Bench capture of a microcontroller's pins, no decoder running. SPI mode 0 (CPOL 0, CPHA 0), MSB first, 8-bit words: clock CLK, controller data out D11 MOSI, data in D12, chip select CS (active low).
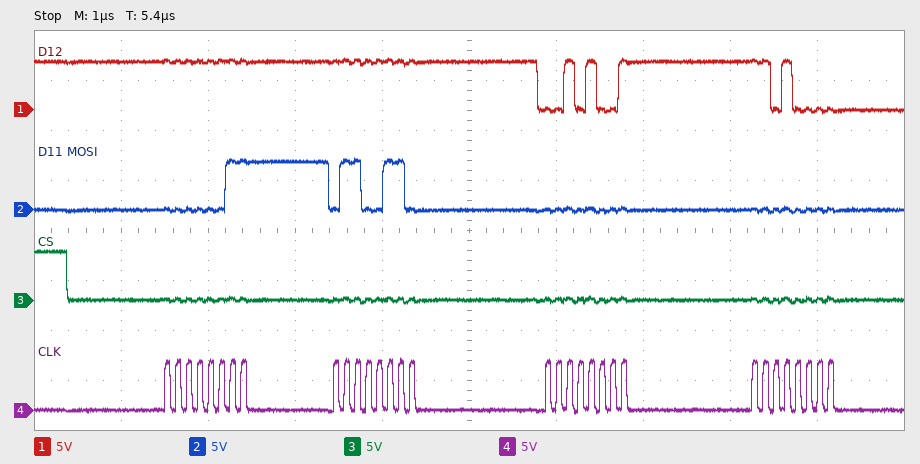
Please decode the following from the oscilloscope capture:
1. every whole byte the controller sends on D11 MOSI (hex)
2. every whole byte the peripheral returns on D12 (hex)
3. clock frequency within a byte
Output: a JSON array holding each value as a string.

["03 66 00 00", "FF FF 29 D0", "8 MHz"]
